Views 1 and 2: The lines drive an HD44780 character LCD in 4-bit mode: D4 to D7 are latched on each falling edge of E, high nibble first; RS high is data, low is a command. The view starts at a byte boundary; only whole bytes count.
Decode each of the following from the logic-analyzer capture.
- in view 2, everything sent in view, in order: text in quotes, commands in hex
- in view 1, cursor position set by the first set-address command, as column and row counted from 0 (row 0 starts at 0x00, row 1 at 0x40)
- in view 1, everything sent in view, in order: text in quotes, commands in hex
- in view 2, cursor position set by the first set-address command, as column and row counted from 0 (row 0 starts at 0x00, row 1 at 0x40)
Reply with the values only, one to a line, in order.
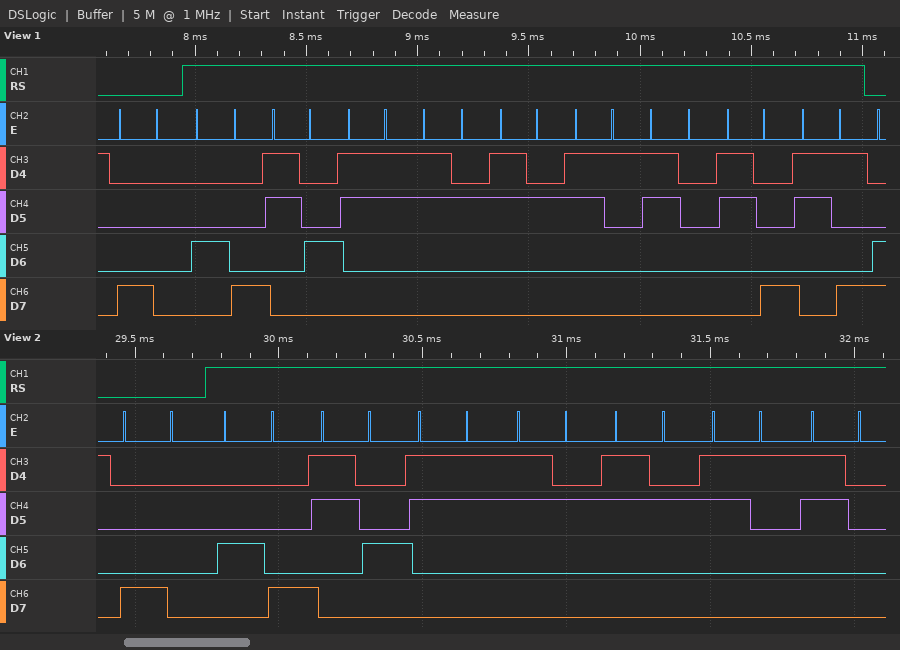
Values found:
0x80 "H432210"
column 0, row 0
0x80 "H43221089"
column 0, row 0
